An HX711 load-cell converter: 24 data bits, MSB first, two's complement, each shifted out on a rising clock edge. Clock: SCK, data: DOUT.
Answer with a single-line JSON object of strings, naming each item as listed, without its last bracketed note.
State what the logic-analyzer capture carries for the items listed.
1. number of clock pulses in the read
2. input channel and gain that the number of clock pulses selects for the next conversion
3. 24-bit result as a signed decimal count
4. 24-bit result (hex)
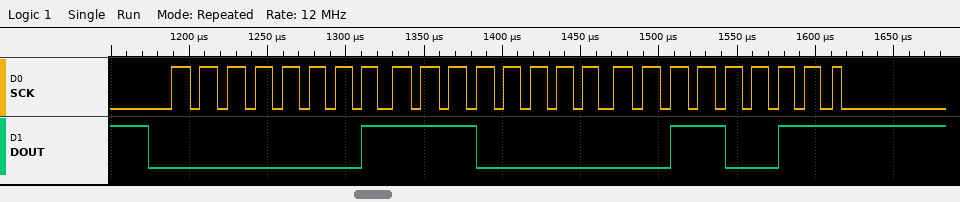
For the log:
{"number of clock pulses in the read": "25", "input channel and gain that the number of clock pulses selects for the next conversion": "channel A, gain 128", "24-bit result as a signed decimal count": "122931", "24-bit result": "0x01E033"}
